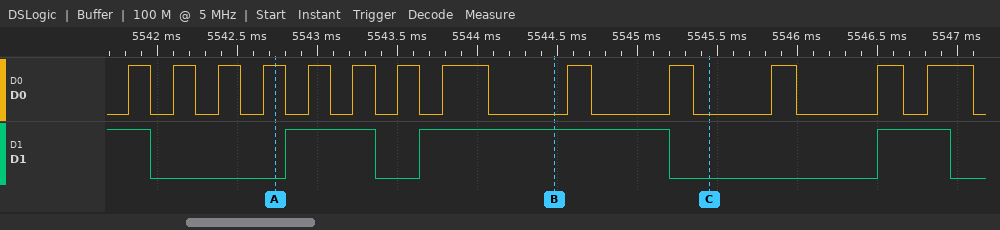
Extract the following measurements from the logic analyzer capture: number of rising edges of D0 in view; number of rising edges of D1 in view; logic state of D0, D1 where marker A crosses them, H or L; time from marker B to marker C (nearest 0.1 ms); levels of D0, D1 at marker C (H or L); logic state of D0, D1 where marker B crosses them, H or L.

13
3
D0=H, D1=L
1 ms
D0=L, D1=L
D0=L, D1=H
